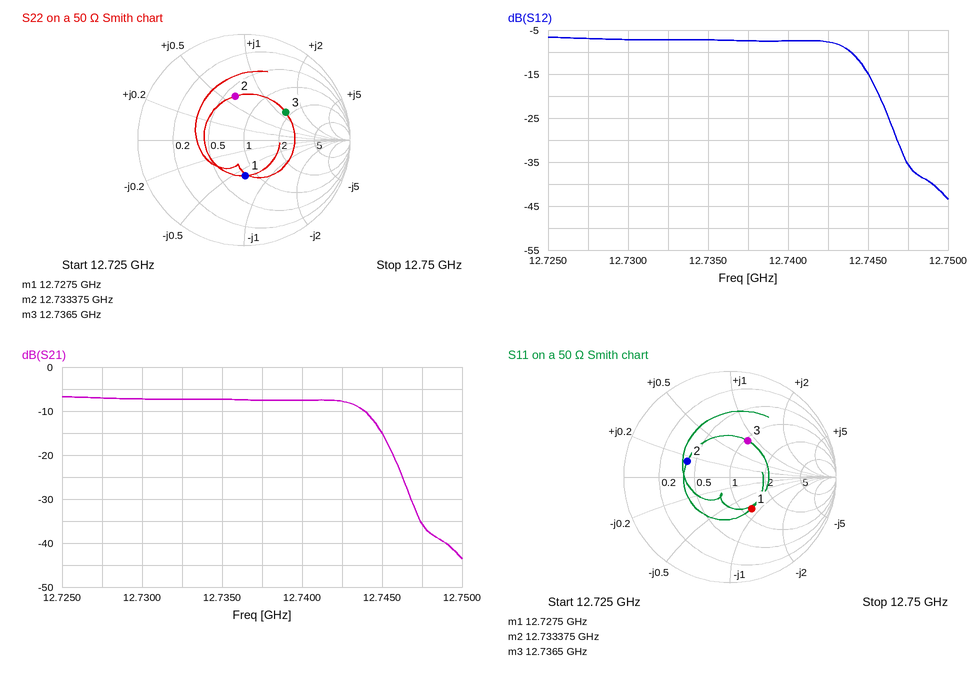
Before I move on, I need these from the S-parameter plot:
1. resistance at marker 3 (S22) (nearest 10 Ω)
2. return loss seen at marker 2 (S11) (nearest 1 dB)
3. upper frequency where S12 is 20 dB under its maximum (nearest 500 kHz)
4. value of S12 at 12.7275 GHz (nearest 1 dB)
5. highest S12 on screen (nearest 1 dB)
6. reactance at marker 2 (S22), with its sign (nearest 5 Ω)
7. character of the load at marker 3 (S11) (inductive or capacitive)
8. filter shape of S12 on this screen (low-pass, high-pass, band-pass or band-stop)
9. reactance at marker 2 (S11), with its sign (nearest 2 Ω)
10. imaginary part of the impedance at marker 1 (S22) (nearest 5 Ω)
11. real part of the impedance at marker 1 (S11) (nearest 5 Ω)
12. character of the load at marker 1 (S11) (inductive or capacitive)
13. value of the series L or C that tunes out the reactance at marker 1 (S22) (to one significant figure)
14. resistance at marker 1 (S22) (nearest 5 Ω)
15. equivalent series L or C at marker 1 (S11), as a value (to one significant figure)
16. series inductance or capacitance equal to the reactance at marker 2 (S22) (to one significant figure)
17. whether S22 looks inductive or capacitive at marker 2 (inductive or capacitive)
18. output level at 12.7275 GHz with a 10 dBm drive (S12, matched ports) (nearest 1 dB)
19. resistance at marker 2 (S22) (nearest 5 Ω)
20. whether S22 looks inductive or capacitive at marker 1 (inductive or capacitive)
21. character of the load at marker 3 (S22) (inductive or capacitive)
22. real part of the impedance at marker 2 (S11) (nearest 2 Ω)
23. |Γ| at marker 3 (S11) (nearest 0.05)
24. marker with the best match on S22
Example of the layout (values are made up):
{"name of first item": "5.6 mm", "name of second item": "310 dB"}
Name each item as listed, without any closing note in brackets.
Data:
{"resistance at marker 3 (S22)": "90 Ω", "return loss seen at marker 2 (S11)": "7 dB", "upper frequency where S12 is 20 dB under its maximum": "12.7465 GHz", "value of S12 at 12.7275 GHz": "-7 dB", "highest S12 on screen": "-7 dB", "reactance at marker 2 (S22), with its sign": "+30 Ω", "character of the load at marker 3 (S11)": "inductive", "filter shape of S12 on this screen": "low-pass", "reactance at marker 2 (S11), with its sign": "+8 Ω", "imaginary part of the impedance at marker 1 (S22)": "-30 Ω", "real part of the impedance at marker 1 (S11)": "60 Ω", "character of the load at marker 1 (S11)": "capacitive", "value of the series L or C that tunes out the reactance at marker 1 (S22)": "400 pH", "resistance at marker 1 (S22)": "40 Ω", "equivalent series L or C at marker 1 (S11), as a value": "300 fF", "series inductance or capacitance equal to the reactance at marker 2 (S22)": "400 pH", "whether S22 looks inductive or capacitive at marker 2": "inductive", "output level at 12.7275 GHz with a 10 dBm drive (S12, matched ports)": "3 dBm", "resistance at marker 2 (S22)": "30 Ω", "whether S22 looks inductive or capacitive at marker 1": "capacitive", "character of the load at marker 3 (S22)": "inductive", "real part of the impedance at marker 2 (S11)": "20 Ω", "|Γ| at marker 3 (S11)": "0.40", "marker with the best match on S22": "marker 1"}
